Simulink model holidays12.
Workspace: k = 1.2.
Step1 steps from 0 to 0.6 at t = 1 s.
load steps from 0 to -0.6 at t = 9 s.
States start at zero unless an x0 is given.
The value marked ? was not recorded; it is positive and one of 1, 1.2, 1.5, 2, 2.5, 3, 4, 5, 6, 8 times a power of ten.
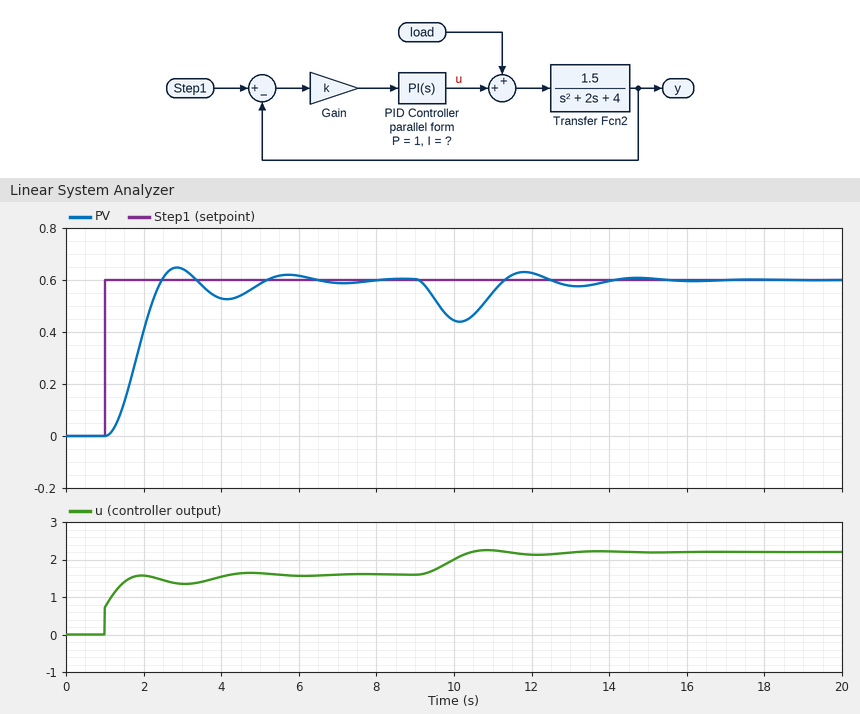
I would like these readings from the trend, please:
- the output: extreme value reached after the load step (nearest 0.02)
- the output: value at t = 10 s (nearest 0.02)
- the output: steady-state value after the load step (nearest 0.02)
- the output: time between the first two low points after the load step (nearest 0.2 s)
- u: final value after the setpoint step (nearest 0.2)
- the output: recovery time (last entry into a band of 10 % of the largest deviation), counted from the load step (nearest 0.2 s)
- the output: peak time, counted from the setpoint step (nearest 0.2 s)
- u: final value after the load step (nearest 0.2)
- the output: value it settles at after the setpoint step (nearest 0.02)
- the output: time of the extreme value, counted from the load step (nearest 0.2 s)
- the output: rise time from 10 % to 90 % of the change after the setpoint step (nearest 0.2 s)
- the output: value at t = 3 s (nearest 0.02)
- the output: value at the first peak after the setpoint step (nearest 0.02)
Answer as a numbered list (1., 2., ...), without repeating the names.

1. 0.44
2. 0.44
3. 0.60
4. 3.0 s
5. 1.6
6. 4.6 s
7. 1.8 s
8. 2.2
9. 0.60
10. 1.2 s
11. 1.0 s
12. 0.64
13. 0.64
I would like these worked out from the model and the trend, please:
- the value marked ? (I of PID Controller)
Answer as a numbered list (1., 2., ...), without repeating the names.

1. 2.5
